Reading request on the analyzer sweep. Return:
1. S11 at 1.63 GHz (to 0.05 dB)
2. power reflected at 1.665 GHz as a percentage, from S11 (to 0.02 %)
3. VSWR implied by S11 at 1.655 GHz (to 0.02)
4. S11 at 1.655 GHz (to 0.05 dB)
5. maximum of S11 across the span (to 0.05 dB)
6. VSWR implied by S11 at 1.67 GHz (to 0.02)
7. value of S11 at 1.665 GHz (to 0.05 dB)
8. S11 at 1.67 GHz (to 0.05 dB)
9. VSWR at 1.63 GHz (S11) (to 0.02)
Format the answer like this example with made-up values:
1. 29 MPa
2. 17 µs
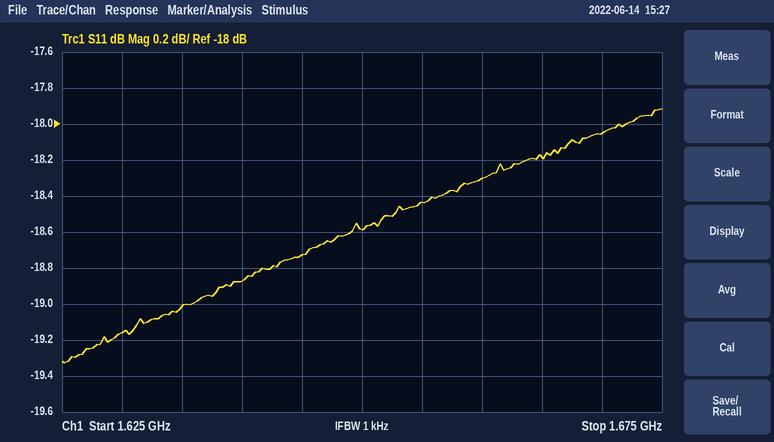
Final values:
1. -19.15 dB
2. 1.52 %
3. 1.28
4. -18.45 dB
5. -17.90 dB
6. 1.28
7. -18.20 dB
8. -18.05 dB
9. 1.24
